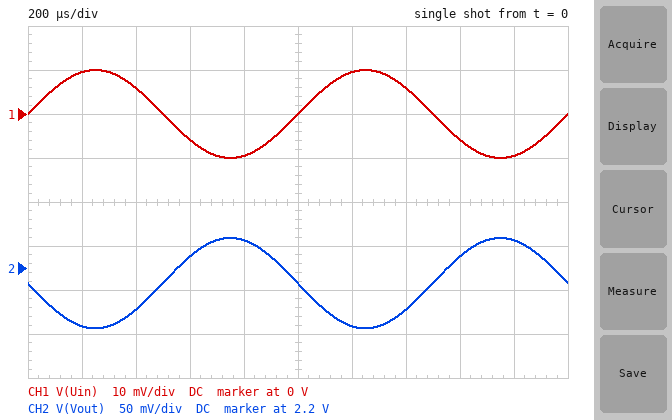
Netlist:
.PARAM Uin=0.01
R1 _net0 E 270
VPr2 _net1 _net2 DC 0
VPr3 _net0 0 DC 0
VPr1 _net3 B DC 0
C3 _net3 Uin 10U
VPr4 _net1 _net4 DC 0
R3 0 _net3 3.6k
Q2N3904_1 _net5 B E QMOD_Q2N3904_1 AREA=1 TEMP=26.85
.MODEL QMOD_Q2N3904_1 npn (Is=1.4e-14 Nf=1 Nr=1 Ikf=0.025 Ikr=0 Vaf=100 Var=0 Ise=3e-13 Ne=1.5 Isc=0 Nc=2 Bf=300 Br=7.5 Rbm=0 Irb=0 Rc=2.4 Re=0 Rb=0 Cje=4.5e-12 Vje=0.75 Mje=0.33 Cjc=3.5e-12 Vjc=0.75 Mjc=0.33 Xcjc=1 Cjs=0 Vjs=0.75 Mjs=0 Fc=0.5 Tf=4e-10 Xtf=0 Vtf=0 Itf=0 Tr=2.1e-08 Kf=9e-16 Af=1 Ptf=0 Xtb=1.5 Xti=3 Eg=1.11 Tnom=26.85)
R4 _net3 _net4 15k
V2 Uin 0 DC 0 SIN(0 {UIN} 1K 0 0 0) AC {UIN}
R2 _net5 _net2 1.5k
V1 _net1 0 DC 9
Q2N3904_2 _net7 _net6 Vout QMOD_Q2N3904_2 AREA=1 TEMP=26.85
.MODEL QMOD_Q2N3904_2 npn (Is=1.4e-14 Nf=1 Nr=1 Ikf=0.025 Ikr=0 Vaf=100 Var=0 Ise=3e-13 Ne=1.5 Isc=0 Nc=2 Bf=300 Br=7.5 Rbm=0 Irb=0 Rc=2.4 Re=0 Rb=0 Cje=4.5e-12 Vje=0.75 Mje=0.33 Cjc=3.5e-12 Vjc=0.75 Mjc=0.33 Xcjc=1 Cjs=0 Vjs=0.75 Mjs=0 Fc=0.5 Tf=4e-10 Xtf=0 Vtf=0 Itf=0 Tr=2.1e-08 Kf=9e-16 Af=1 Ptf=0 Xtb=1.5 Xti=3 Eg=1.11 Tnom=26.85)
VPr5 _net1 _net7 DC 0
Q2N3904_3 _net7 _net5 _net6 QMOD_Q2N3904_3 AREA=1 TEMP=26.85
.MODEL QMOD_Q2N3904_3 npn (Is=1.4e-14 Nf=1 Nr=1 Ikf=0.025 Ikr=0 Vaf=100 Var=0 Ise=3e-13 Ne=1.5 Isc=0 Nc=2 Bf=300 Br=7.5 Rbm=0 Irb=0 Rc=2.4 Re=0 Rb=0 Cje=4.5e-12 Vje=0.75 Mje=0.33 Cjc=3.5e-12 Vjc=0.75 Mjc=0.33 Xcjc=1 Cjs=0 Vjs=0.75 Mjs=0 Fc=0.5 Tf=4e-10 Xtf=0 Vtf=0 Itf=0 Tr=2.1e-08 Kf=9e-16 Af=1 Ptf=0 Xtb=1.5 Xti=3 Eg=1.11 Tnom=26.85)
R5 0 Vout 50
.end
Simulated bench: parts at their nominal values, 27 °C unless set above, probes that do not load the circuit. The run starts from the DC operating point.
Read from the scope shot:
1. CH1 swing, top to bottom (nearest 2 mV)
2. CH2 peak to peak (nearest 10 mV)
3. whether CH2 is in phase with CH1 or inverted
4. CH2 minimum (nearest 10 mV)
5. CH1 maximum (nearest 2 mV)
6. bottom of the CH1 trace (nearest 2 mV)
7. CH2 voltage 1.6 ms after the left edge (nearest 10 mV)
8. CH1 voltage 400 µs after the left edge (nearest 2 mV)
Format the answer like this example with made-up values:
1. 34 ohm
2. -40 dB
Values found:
1. 20 mV
2. 100 mV
3. inverted
4. 2.13 V
5. 10 mV
6. -10 mV
7. 2.21 V
8. 6 mV
